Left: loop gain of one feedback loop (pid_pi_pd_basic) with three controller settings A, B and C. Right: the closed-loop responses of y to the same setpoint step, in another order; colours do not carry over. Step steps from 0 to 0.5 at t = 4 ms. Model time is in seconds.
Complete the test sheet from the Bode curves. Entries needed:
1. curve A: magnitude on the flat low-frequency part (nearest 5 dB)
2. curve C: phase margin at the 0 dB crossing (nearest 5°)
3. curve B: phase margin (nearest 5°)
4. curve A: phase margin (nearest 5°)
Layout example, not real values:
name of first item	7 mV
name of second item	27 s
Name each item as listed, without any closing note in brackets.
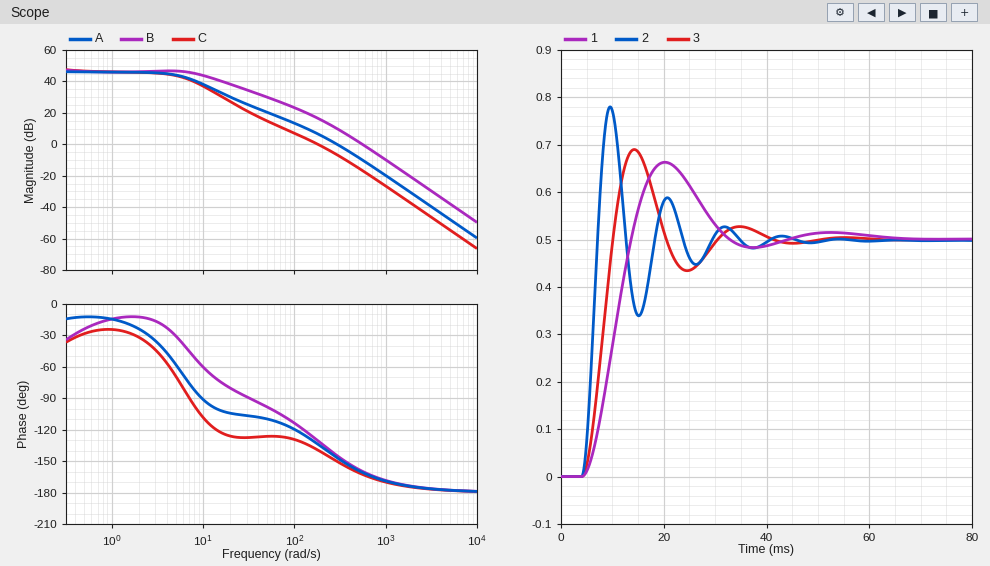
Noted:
curve A: magnitude on the flat low-frequency part	45 dB
curve C: phase margin at the 0 dB crossing	40°
curve B: phase margin	20°
curve A: phase margin	35°
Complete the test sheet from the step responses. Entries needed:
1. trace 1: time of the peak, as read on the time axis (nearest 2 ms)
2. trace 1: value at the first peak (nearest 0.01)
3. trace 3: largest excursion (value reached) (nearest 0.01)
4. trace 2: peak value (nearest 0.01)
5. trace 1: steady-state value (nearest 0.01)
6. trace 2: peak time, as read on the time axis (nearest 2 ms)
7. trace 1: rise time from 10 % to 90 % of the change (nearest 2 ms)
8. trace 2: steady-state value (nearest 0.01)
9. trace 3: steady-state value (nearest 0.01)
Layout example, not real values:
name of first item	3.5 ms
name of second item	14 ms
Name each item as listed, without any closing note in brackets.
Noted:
trace 1: time of the peak, as read on the time axis	20 ms
trace 1: value at the first peak	0.66
trace 3: largest excursion (value reached)	0.69
trace 2: peak value	0.78
trace 1: steady-state value	0.50
trace 2: peak time, as read on the time axis	10 ms
trace 1: rise time from 10 % to 90 % of the change	6 ms
trace 2: steady-state value	0.50
trace 3: steady-state value	0.50
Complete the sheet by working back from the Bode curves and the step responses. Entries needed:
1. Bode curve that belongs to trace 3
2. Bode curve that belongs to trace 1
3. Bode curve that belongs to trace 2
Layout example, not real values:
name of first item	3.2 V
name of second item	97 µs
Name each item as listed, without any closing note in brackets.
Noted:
Bode curve that belongs to trace 3	A
Bode curve that belongs to trace 1	C
Bode curve that belongs to trace 2	B
